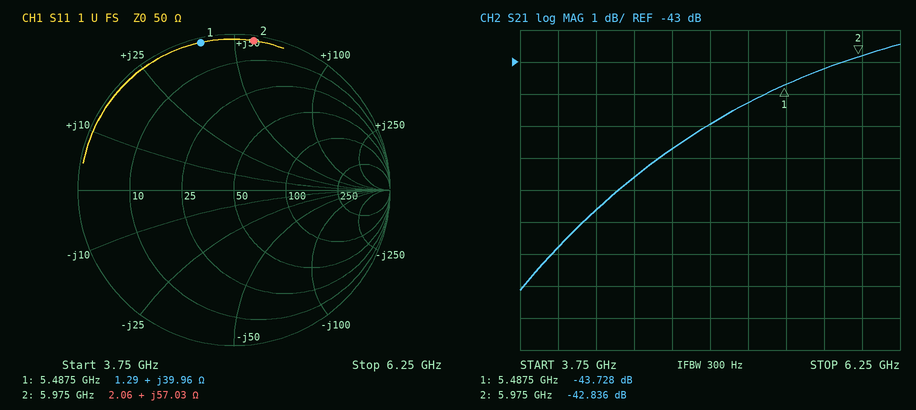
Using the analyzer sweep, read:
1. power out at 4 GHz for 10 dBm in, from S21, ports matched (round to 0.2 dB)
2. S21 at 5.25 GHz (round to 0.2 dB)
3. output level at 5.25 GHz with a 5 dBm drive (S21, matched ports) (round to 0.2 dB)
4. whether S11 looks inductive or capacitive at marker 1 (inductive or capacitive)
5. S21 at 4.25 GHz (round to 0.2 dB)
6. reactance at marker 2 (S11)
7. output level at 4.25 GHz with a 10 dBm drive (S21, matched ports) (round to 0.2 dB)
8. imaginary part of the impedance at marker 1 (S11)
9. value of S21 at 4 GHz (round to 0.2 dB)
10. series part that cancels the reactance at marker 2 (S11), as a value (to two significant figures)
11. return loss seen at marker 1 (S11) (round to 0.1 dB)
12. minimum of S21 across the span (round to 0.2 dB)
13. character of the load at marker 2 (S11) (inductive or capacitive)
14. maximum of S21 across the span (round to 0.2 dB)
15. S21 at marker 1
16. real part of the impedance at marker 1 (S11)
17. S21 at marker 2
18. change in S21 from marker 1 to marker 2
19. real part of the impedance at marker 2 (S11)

-38.8 dBm
-44.2 dB
-39.2 dBm
inductive
-47.6 dB
+57.03 Ω
-37.6 dBm
+39.96 Ω
-48.8 dB
470 fF
0.3 dB
-50.2 dB
inductive
-42.4 dB
-43.728 dB
1.29 Ω
-42.836 dB
0.892 dB
2.06 Ω
